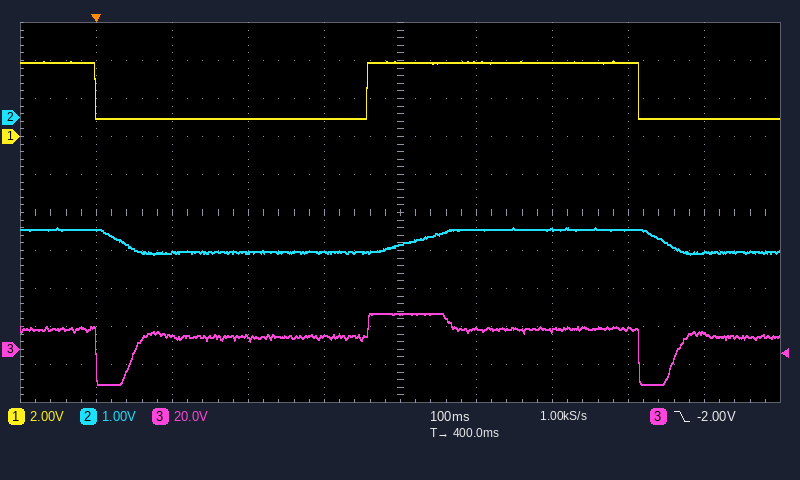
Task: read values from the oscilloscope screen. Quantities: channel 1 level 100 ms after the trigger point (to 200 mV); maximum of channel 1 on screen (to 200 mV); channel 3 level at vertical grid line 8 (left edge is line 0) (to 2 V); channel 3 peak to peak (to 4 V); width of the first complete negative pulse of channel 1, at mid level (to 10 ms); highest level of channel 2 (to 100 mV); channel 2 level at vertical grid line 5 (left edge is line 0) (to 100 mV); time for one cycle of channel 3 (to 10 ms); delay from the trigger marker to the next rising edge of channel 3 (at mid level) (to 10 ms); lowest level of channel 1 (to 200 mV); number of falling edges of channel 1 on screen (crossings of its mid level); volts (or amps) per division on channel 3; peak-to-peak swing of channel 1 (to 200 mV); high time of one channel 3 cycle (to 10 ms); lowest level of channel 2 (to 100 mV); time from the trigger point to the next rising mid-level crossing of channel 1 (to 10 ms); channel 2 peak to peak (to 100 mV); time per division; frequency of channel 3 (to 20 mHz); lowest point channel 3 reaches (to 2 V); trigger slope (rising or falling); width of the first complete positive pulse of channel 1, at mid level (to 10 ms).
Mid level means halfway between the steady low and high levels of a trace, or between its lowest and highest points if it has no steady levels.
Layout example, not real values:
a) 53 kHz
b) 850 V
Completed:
a) 1.0 V
b) 4.0 V
c) 10 V
d) 36 V
e) 360 ms
f) -2.9 V
g) -3.3 V
h) 710 ms
i) 50 ms
j) 1.0 V
k) 2
l) 20 V
m) 3.0 V
n) 660 ms
o) -3.6 V
p) 360 ms
q) 700 mV
r) 100 ms
s) 1.40 Hz
t) -18 V
u) falling
v) 360 ms
